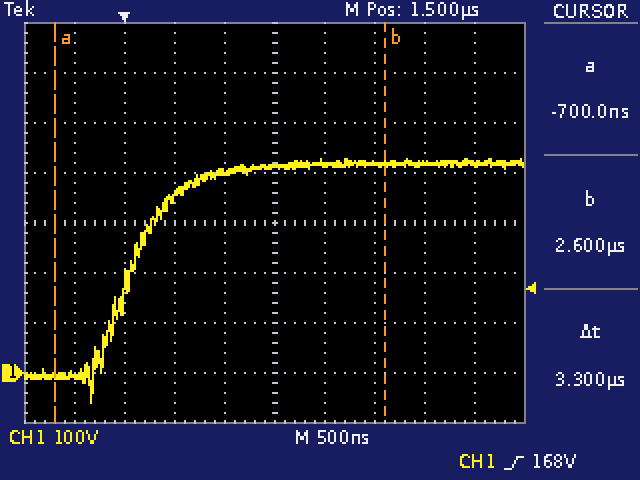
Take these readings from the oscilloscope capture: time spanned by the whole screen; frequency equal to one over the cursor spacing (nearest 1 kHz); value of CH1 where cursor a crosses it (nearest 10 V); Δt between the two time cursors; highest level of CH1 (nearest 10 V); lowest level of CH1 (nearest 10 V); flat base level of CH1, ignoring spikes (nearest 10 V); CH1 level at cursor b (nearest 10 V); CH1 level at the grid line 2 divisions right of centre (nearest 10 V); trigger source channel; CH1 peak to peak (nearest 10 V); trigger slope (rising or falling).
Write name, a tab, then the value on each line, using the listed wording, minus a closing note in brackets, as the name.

time spanned by the whole screen	5 µs
frequency equal to one over the cursor spacing	303 kHz
value of CH1 where cursor a crosses it	-10 V
Δt between the two time cursors	3.3 µs
highest level of CH1	430 V
lowest level of CH1	-60 V
flat base level of CH1, ignoring spikes	-10 V
CH1 level at cursor b	420 V
CH1 level at the grid line 2 divisions right of centre	420 V
trigger source channel	CH1
CH1 peak to peak	490 V
trigger slope	rising
